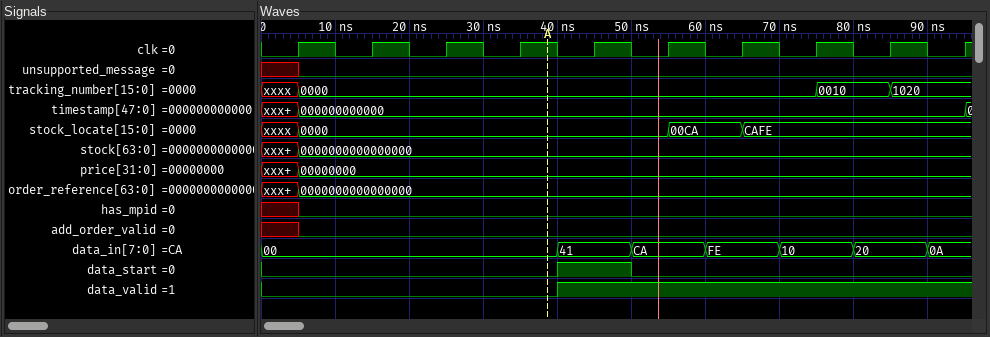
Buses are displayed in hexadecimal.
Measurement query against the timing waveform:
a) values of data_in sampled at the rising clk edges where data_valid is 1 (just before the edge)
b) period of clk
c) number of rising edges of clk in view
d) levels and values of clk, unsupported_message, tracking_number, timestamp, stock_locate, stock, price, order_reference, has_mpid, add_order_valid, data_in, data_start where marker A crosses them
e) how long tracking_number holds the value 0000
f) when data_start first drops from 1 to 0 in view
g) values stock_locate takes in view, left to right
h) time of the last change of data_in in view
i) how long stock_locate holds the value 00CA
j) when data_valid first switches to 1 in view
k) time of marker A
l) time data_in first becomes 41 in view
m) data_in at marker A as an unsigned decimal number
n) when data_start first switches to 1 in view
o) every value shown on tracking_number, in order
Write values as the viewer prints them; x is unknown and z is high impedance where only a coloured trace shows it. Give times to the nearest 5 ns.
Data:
41, CA, FE, 10, 20, 0A
10 ns
10
clk=1, unsupported_message=0, tracking_number=0000, timestamp=000000000000, stock_locate=0000, stock=0000000000000000, price=00000000, order_reference=0000000000000000, has_mpid=0, add_order_valid=0, data_in=00, data_start=0
70 ns
50 ns
xxxx, 0000, 00CA, CAFE
90 ns
10 ns
40 ns
40 ns
40 ns
0
40 ns
xxxx, 0000, 0010, 1020
